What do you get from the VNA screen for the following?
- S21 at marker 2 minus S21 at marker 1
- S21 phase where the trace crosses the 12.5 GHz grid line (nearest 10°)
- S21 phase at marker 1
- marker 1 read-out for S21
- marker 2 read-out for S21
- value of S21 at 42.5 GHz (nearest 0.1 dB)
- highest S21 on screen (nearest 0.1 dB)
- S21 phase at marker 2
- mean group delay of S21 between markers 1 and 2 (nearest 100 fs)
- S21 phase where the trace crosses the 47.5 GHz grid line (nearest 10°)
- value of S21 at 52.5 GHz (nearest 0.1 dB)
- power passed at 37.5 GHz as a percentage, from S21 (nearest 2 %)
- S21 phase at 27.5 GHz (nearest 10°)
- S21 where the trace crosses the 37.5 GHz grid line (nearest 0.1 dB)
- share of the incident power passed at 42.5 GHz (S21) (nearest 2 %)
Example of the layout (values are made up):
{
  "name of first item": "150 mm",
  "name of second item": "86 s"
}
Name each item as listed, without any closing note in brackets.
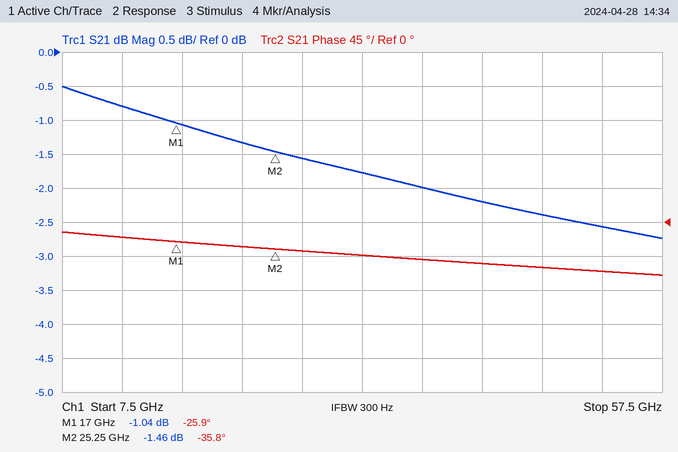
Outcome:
{
  "S21 at marker 2 minus S21 at marker 1": "-0.42 dB",
  "S21 phase where the trace crosses the 12.5 GHz grid line": "-20°",
  "S21 phase at marker 1": "-25.9°",
  "marker 1 read-out for S21": "-1.04 dB",
  "marker 2 read-out for S21": "-1.46 dB",
  "value of S21 at 42.5 GHz": "-2.2 dB",
  "highest S21 on screen": "-0.5 dB",
  "S21 phase at marker 2": "-35.8°",
  "mean group delay of S21 between markers 1 and 2": "3.3 ps",
  "S21 phase where the trace crosses the 47.5 GHz grid line": "-60°",
  "value of S21 at 52.5 GHz": "-2.6 dB",
  "power passed at 37.5 GHz as a percentage, from S21": "64 %",
  "S21 phase at 27.5 GHz": "-40°",
  "S21 where the trace crosses the 37.5 GHz grid line": "-2.0 dB",
  "share of the incident power passed at 42.5 GHz (S21)": "60 %"
}
